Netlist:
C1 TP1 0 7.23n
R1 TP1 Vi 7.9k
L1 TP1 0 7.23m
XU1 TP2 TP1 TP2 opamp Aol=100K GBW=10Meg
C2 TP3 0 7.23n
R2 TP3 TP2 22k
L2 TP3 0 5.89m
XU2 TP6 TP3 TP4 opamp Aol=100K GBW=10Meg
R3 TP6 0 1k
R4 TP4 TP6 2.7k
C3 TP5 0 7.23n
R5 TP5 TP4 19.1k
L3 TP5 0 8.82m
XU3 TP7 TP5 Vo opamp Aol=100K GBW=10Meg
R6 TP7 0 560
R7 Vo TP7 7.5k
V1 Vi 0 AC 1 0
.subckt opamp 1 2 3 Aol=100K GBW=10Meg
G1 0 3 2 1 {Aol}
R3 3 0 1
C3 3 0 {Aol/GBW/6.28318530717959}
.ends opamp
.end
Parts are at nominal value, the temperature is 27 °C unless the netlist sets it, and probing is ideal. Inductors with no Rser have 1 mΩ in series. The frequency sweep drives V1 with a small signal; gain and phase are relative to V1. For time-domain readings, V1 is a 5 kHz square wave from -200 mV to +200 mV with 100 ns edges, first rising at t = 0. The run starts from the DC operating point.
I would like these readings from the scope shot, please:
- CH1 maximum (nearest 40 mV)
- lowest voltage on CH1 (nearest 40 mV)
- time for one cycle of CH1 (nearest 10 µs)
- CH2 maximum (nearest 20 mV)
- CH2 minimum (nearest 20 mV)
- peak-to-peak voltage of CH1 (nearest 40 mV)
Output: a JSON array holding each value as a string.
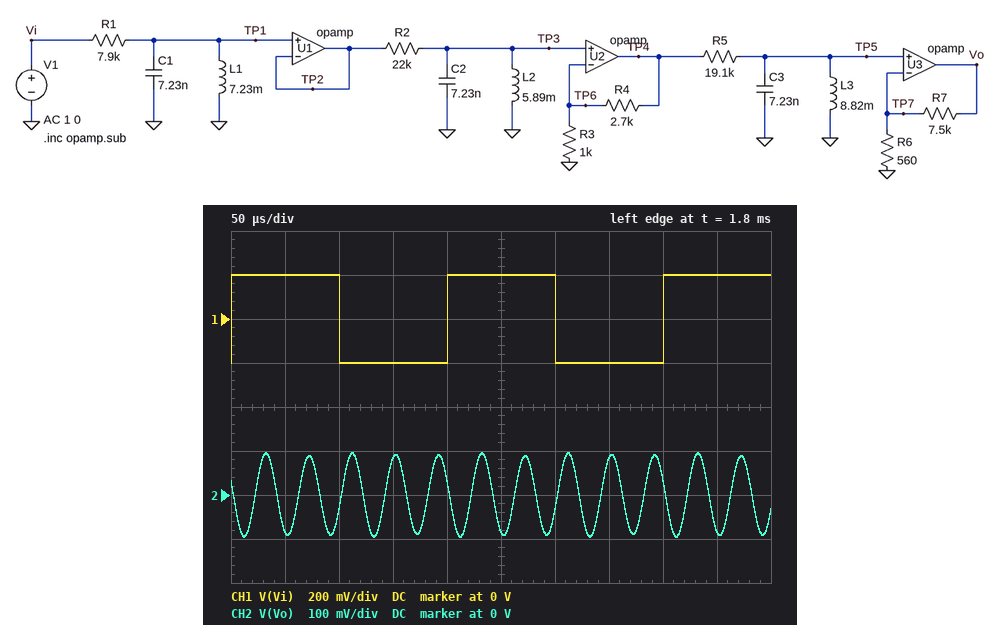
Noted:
["200 mV", "-200 mV", "200 µs", "100 mV", "-100 mV", "400 mV"]
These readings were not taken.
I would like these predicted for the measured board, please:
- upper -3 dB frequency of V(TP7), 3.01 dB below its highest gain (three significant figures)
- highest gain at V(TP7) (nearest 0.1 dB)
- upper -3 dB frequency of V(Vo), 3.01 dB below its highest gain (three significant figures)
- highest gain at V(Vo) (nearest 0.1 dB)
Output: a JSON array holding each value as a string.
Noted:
["24.7 kHz", "-11.0 dB", "24.7 kHz", "12.2 dB"]
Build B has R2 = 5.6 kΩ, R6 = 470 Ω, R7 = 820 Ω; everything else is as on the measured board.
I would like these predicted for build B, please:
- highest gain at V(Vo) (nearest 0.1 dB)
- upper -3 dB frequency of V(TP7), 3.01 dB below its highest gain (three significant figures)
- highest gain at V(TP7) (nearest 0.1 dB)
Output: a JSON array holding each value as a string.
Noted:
["6.6 dB", "22.6 kHz", "-2.2 dB"]
